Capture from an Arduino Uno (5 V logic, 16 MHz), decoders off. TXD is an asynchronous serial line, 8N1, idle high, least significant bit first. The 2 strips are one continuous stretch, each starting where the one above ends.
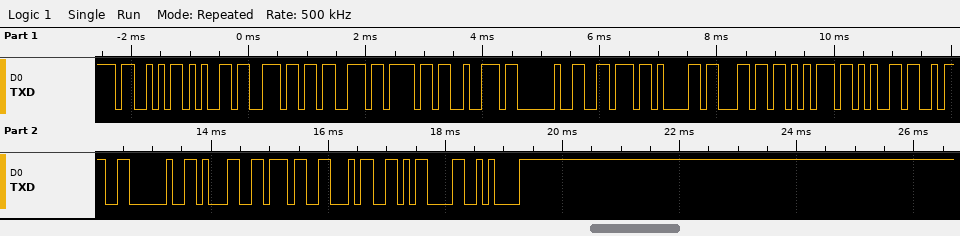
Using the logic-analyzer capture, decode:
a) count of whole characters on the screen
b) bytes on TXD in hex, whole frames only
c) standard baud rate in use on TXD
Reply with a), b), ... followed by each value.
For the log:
a) 19
b) 0x53 0x65 0x6E 0x73 0x6F 0x72 0x20 0x76 0x61 0x6C 0x75 0x65 0x3A 0x20 0x31 0x37 0x34 0x0D 0x0A
c) 9600 baud
